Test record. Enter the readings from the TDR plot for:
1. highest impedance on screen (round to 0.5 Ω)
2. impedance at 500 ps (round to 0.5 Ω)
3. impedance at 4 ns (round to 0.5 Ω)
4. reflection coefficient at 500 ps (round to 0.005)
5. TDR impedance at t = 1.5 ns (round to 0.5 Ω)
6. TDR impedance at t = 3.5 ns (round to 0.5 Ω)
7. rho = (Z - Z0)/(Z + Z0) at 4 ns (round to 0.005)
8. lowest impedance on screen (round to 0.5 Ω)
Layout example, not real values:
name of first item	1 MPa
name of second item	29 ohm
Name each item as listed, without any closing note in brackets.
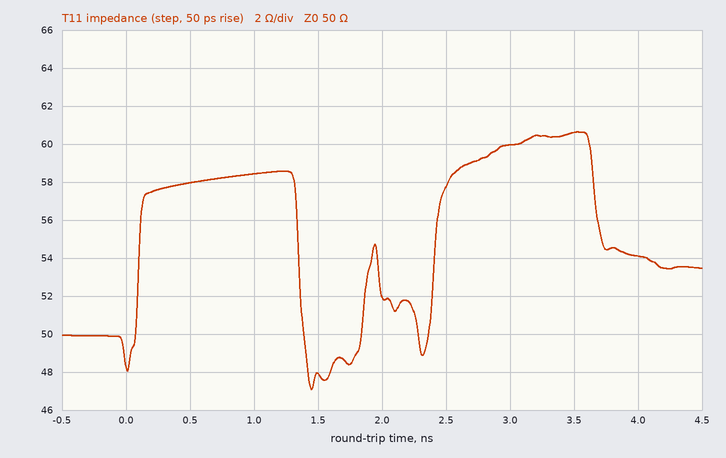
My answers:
highest impedance on screen	60.5 Ω
impedance at 500 ps	58.0 Ω
impedance at 4 ns	54.0 Ω
reflection coefficient at 500 ps	+0.075
TDR impedance at t = 1.5 ns	48.0 Ω
TDR impedance at t = 3.5 ns	60.5 Ω
rho = (Z - Z0)/(Z + Z0) at 4 ns	+0.040
lowest impedance on screen	47.0 Ω
